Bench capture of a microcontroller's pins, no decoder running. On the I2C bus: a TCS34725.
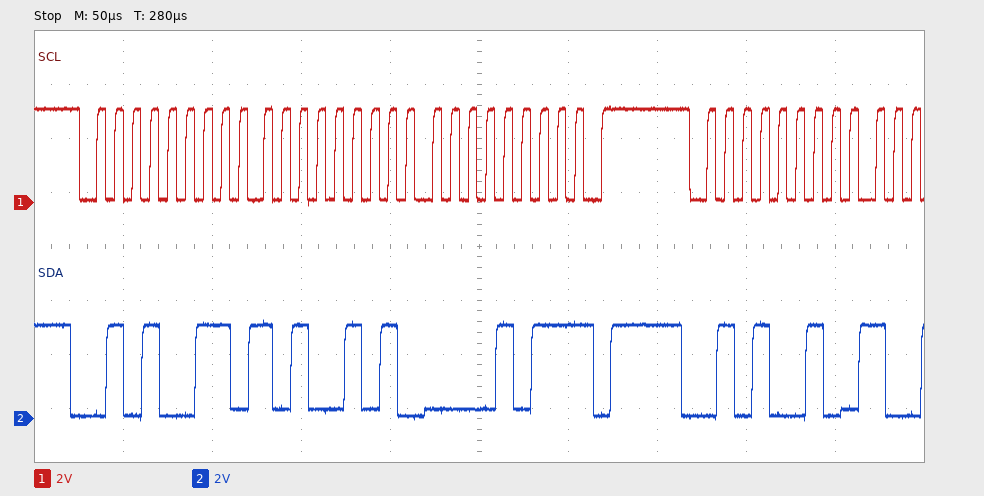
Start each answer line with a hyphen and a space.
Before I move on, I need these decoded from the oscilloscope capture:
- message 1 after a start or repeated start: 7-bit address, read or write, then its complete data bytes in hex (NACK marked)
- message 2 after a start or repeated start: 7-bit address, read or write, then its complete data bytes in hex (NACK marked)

- 0x29 read: A5 0B NACK
- 0x29 write
